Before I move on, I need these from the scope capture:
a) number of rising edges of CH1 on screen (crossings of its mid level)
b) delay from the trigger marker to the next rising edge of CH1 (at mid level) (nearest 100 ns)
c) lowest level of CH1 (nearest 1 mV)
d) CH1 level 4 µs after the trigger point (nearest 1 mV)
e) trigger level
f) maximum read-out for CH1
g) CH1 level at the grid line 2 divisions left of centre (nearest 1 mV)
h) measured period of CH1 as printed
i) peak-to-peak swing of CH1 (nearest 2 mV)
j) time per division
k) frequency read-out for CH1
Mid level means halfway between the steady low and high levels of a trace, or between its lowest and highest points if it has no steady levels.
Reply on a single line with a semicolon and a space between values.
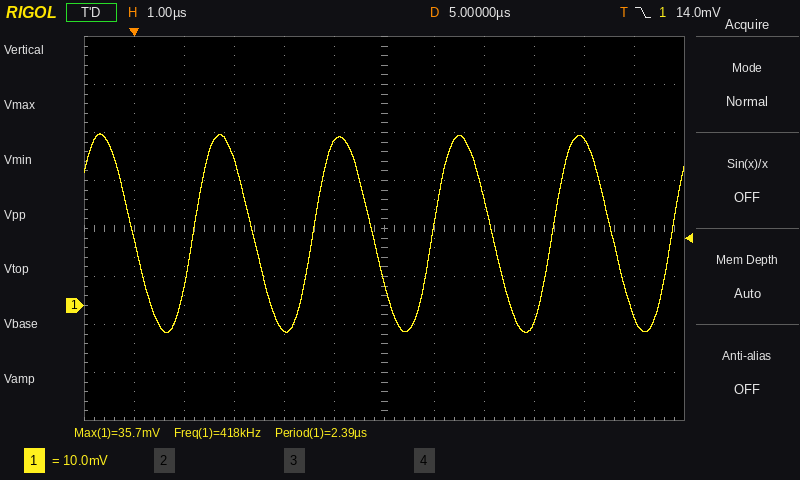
5; 1.2 µs; -6 mV; 34 mV; 14.0 mV; 35.7 mV; -5 mV; 2.39 µs; 42 mV; 1 µs; 418 kHz
